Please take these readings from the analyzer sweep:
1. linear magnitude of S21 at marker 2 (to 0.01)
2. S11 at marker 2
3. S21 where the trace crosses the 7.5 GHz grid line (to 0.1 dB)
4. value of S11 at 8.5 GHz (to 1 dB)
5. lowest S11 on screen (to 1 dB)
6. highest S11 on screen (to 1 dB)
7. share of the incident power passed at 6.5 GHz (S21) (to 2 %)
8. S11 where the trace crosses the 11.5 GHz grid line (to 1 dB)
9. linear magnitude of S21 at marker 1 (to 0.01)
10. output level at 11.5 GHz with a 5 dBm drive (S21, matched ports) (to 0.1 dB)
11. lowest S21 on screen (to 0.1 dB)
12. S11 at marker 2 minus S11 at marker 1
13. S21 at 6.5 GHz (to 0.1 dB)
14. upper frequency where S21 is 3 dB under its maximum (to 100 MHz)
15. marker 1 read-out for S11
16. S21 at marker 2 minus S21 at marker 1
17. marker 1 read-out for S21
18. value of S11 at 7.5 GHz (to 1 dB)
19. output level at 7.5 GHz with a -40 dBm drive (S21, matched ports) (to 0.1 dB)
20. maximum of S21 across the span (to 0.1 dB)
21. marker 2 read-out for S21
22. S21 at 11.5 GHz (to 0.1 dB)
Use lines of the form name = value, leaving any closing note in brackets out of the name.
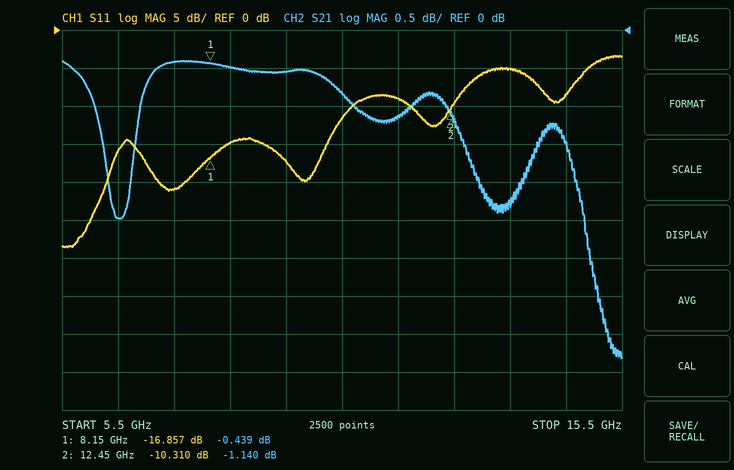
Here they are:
linear magnitude of S21 at marker 2 = 0.88
S11 at marker 2 = -10.310 dB
S21 where the trace crosses the 7.5 GHz grid line = -0.4 dB
value of S11 at 8.5 GHz = -15 dB
lowest S11 on screen = -29 dB
highest S11 on screen = -3 dB
share of the incident power passed at 6.5 GHz (S21) = 56 %
S11 where the trace crosses the 11.5 GHz grid line = -9 dB
linear magnitude of S21 at marker 1 = 0.95
output level at 11.5 GHz with a 5 dBm drive (S21, matched ports) = 3.9 dBm
lowest S21 on screen = -4.3 dB
S11 at marker 2 minus S11 at marker 1 = 6.547 dB
S21 at 6.5 GHz = -2.5 dB
upper frequency where S21 is 3 dB under its maximum = 15.0 GHz
marker 1 read-out for S11 = -16.857 dB
S21 at marker 2 minus S21 at marker 1 = -0.701 dB
marker 1 read-out for S21 = -0.439 dB
value of S11 at 7.5 GHz = -21 dB
output level at 7.5 GHz with a -40 dBm drive (S21, matched ports) = -40.4 dBm
maximum of S21 across the span = -0.4 dB
marker 2 read-out for S21 = -1.140 dB
S21 at 11.5 GHz = -1.1 dB
